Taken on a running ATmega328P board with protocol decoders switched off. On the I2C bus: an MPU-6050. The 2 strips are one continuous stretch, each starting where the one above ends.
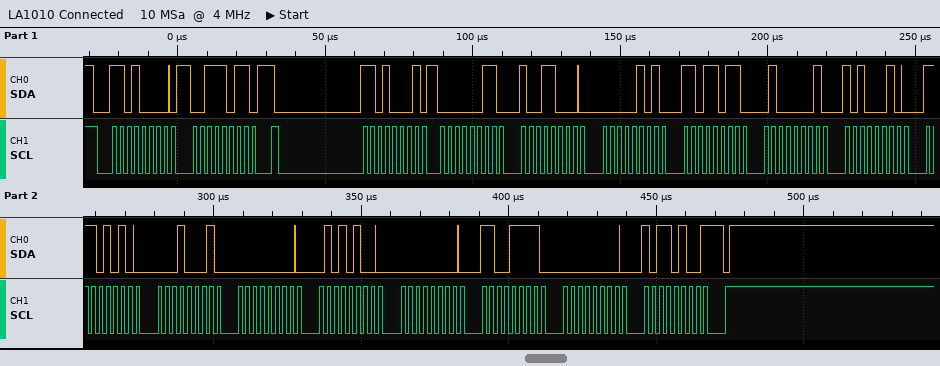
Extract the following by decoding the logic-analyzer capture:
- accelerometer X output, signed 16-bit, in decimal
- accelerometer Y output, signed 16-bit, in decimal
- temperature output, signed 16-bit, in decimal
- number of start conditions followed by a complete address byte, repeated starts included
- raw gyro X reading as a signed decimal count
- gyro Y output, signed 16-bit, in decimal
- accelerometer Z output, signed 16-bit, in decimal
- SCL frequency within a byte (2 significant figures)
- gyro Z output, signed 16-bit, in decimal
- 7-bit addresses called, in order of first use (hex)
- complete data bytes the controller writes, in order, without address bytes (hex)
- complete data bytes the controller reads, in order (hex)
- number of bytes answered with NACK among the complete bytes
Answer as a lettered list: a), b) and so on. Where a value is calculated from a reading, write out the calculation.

a) 0x0398 = 920
b) 0x05DB = 1499
c) 0xEA11 = -5615
d) 2
e) 0x0054 = 84
f) 0x00CF = 207
g) 0x41A2 = 16802
h) 400 kHz
i) 0x00B4 = 180
j) 0x68
k) 3B
l) 03 98 05 DB 41 A2 EA 11 00 54 00 CF 00 B4
m) 1
